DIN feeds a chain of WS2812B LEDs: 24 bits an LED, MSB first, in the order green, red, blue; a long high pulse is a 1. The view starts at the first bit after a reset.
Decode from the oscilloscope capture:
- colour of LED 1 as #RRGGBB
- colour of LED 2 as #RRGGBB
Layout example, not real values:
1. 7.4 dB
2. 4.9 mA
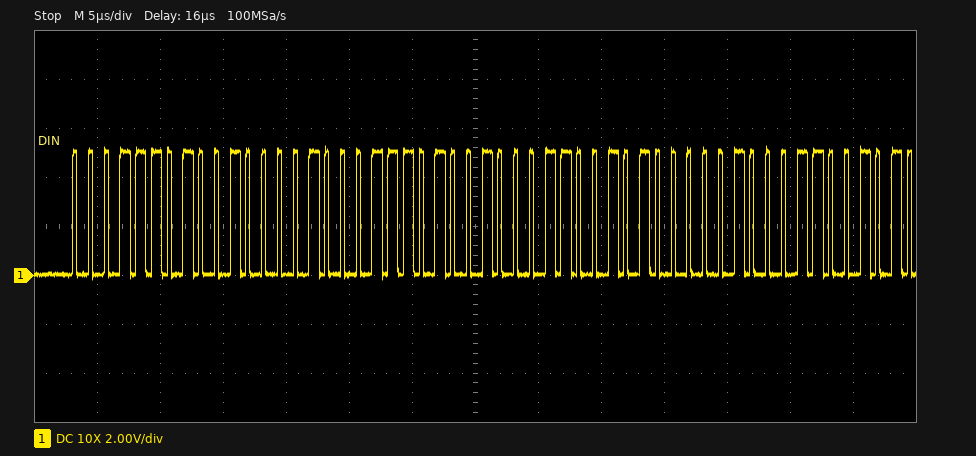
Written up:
1. #211D1D
2. #282323
